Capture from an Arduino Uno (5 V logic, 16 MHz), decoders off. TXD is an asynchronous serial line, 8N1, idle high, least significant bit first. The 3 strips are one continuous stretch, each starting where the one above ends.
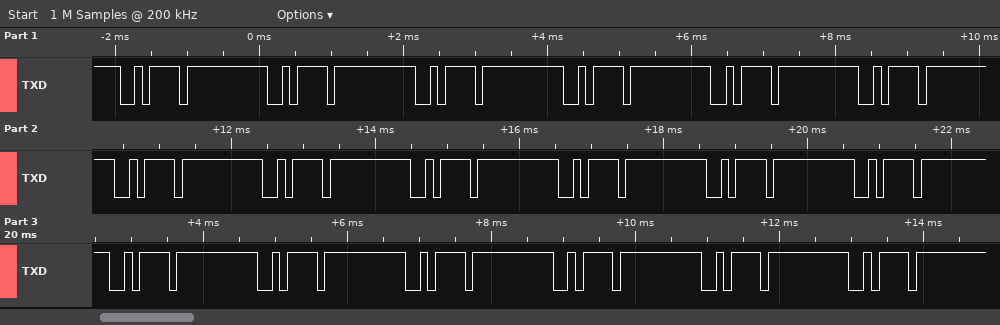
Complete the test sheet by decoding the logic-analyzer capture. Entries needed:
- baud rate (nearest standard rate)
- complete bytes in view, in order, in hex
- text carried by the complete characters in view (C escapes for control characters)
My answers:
9600 baud
7A 7A 7A 7A 7A 7A 7A 7A 7A 7A 7A 7A 7A 7A 7A 7A 7A 7A
"zzzzzzzzzzzzzzzzzz"
